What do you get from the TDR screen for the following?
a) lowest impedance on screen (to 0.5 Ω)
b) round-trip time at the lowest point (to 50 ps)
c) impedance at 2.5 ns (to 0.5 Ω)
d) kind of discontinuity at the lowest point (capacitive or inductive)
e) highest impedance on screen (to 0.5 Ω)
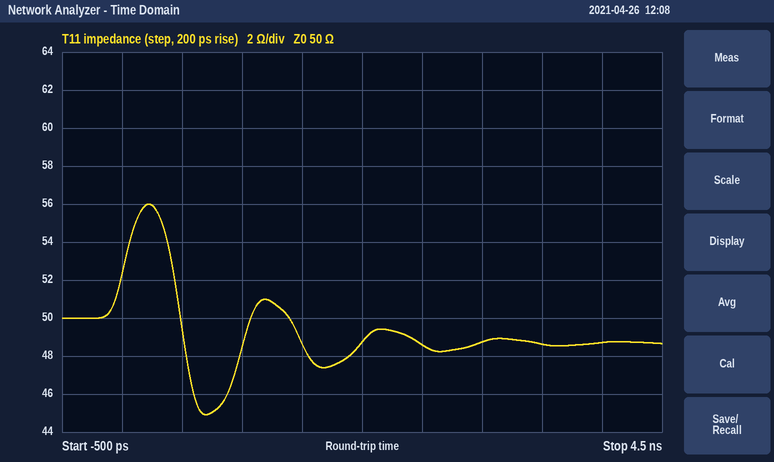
45.0 Ω
700 ps
48.5 Ω
capacitive
56.0 Ω
